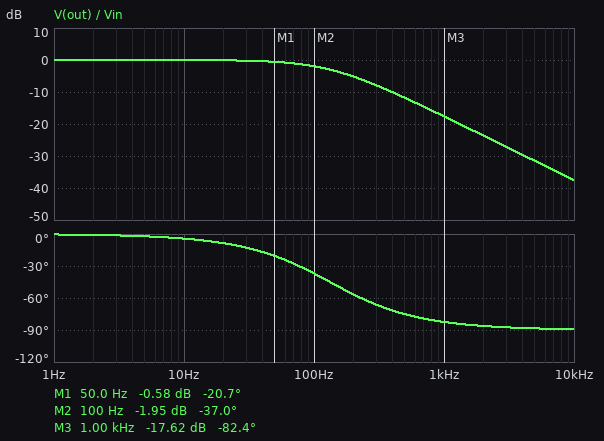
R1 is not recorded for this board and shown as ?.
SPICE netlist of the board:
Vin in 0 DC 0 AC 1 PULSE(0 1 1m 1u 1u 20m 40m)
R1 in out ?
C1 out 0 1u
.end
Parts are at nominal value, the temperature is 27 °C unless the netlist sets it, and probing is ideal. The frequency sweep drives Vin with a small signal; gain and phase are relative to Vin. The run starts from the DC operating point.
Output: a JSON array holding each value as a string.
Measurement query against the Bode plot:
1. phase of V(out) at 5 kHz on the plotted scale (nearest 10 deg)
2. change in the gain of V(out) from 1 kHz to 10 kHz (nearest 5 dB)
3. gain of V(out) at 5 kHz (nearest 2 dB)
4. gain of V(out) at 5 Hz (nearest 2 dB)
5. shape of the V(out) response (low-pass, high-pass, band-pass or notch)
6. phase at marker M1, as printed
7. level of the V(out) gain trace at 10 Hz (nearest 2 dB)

["-90 deg", "-20 dB", "-32 dB", "0 dB", "low-pass", "-20.7 deg", "0 dB"]
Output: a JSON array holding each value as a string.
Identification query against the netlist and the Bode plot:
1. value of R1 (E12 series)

["1.2 kΩ"]
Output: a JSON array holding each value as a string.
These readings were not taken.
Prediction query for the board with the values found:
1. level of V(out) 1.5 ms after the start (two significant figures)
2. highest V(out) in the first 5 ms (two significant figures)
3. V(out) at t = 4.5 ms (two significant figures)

["340 mV", "960 mV", "950 mV"]
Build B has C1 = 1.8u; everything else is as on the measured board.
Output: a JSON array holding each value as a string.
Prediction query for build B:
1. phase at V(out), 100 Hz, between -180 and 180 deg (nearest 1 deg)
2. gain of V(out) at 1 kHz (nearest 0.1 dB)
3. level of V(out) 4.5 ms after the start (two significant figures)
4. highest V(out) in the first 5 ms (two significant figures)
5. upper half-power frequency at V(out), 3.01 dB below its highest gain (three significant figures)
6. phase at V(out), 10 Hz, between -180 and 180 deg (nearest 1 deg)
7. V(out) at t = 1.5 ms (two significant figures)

["-54 deg", "-22.7 dB", "800 mV", "840 mV", "73.7 Hz", "-8 deg", "210 mV"]
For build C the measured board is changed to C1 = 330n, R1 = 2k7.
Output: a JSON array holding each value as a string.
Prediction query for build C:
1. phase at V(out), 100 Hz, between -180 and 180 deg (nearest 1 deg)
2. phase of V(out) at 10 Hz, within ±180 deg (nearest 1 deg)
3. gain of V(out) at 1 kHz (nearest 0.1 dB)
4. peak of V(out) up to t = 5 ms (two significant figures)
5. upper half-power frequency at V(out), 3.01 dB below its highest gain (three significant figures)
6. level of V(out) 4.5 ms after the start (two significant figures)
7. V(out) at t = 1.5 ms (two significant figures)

["-29 deg", "-3 deg", "-15.1 dB", "990 mV", "179 Hz", "980 mV", "430 mV"]
